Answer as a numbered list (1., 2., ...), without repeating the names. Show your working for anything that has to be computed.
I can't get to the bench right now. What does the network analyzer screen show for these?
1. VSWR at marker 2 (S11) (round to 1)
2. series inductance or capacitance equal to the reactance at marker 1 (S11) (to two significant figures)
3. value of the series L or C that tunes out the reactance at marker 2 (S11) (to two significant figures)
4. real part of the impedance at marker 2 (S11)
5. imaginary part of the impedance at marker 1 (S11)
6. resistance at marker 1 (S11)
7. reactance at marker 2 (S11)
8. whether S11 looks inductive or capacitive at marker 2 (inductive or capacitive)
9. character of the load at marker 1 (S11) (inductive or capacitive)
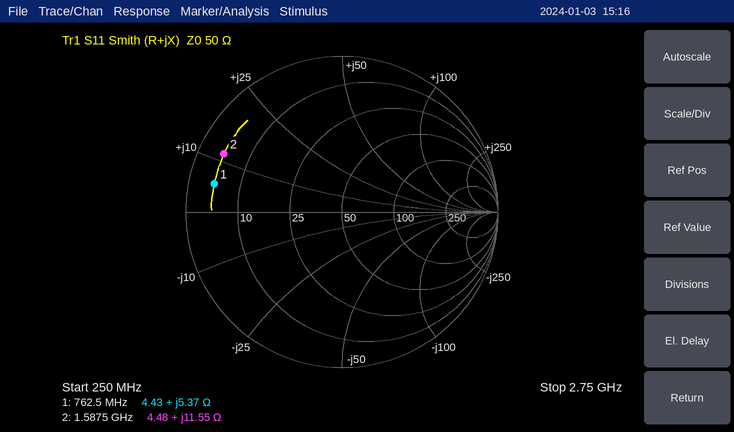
1. 12
2. L = 5.37 Ω/(2π × 762.5 MHz) ≈ 1.1 nH
3. C = 1/(2π × 1.5875 GHz × 11.55 Ω) ≈ 8.7 pF
4. 4.48 Ω
5. +5.37 Ω
6. 4.43 Ω
7. +11.55 Ω
8. inductive
9. inductive
